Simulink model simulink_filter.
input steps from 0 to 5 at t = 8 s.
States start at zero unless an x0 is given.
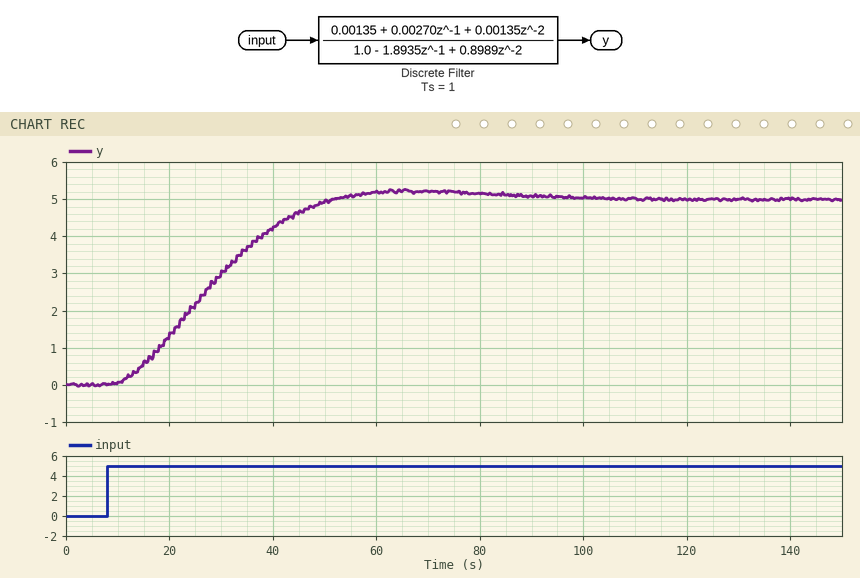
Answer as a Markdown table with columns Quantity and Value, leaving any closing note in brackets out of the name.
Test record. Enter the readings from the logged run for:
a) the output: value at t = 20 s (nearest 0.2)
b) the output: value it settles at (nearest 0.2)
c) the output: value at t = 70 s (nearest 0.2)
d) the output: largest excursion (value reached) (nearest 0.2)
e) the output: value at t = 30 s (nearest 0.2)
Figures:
| Quantity | Value |
|---|---|
| the output: value at t = 20 s | 1.4 |
| the output: value it settles at | 5.0 |
| the output: value at t = 70 s | 5.2 |
| the output: largest excursion (value reached) | 5.2 |
| the output: value at t = 30 s | 3.0 |
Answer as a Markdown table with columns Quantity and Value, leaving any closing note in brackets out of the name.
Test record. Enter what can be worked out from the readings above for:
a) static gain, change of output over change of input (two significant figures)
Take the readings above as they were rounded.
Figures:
| Quantity | Value |
|---|---|
| static gain, change of output over change of input | 1.0 |
